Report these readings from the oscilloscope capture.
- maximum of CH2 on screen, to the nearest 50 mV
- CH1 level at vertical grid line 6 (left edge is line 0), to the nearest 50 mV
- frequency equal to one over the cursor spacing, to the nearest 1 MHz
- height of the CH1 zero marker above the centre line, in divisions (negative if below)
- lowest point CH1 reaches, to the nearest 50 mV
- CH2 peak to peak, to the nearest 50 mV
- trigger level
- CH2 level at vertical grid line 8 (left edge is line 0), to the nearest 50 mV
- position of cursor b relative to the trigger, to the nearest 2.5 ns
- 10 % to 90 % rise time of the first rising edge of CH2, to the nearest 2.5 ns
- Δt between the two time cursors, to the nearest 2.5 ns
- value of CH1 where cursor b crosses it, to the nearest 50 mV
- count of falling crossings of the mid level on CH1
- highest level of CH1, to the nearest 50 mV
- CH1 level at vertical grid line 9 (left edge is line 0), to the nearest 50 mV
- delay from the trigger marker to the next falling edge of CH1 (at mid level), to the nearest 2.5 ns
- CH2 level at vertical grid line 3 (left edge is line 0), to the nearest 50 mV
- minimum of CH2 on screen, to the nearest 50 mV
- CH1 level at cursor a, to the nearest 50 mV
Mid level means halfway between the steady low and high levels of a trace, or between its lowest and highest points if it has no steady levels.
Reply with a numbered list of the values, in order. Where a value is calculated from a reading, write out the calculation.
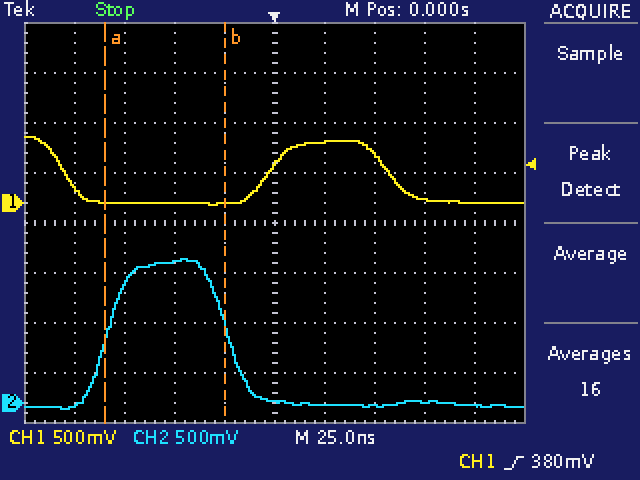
1. 1.45 V
2. 600 mV
3. 1 / 60.0 ns ≈ 17 MHz
4. +0.4 div
5. 0 mV
6. 1.45 V − (-50 mV) = 1.50 V
7. 380 mV
8. 0 mV
9. -25.0 ns
10. 20.0 ns
11. 60.0 ns
12. 0 mV
13. 2
14. 650 mV
15. 0 mV
16. 57.5 ns
17. 1.40 V
18. -50 mV
19. 0 mV
